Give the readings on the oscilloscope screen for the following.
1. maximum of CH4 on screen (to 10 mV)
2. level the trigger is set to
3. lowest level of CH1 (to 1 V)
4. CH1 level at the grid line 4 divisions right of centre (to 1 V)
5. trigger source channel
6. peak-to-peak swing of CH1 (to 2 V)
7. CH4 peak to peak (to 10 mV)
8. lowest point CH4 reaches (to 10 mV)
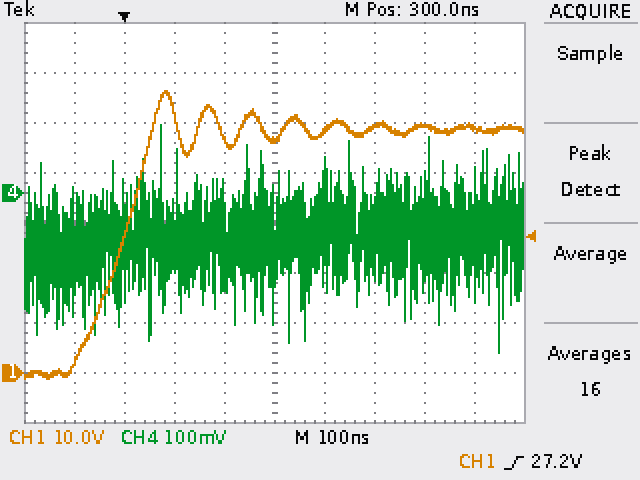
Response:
140 mV
27.2 V
-1 V
49 V
CH1
58 V
460 mV
-320 mV
